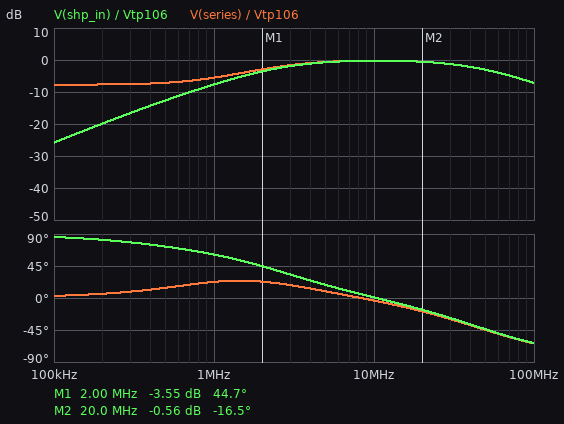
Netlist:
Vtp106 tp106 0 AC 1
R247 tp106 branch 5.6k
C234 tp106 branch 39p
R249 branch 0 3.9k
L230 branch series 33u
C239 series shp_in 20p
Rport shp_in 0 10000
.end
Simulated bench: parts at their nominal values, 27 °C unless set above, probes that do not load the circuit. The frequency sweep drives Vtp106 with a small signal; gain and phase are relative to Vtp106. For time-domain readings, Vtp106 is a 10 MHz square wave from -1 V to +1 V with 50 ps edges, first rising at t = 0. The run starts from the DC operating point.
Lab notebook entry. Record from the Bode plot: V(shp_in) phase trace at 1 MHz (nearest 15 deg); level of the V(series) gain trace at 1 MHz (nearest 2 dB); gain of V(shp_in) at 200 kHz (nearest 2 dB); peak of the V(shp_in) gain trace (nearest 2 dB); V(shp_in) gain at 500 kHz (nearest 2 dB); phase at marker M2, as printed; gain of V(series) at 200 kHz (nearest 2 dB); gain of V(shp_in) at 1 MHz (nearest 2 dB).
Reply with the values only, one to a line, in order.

60 deg
-6 dB
-20 dB
0 dB
-12 dB
-16.5 deg
-8 dB
-8 dB
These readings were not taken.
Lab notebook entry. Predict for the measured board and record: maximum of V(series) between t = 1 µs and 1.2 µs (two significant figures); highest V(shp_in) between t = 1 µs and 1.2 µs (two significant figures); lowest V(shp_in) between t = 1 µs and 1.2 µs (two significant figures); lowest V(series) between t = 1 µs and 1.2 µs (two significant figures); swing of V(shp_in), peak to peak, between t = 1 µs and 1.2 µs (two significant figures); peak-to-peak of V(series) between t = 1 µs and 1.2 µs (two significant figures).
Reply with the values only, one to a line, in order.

1.1 V
1.2 V
-1.2 V
-1.1 V
2.3 V
2.2 V
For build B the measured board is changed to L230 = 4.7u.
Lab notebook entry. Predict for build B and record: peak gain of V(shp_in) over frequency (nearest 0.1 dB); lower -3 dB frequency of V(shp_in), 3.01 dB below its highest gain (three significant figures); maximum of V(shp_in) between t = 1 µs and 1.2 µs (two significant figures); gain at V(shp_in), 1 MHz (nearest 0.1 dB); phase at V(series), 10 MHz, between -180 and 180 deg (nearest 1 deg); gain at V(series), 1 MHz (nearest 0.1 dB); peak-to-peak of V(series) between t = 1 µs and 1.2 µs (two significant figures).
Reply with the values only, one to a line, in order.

0 dB
2.29 MHz
1.3 V
-7.7 dB
6 deg
-5.6 dB
2.4 V
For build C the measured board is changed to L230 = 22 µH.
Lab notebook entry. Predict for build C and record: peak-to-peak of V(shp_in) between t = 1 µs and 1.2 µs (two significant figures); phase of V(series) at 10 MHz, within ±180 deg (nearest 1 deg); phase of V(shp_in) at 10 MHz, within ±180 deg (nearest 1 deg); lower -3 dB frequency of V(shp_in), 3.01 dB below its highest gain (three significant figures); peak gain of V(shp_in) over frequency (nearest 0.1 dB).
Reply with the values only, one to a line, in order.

2.4 V
0 deg
5 deg
2.20 MHz
-0.1 dB
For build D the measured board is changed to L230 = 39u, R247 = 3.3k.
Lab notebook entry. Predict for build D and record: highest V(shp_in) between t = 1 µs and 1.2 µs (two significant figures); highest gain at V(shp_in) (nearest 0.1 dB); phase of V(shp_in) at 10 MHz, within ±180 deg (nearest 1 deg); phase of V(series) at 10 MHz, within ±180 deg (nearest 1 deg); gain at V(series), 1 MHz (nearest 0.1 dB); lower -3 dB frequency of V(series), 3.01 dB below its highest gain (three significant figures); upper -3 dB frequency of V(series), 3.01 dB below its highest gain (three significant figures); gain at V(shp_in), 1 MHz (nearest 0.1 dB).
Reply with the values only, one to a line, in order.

1.1 V
-0.3 dB
-1 deg
-6 deg
-4.8 dB
1.86 MHz
44.4 MHz
-7.0 dB
